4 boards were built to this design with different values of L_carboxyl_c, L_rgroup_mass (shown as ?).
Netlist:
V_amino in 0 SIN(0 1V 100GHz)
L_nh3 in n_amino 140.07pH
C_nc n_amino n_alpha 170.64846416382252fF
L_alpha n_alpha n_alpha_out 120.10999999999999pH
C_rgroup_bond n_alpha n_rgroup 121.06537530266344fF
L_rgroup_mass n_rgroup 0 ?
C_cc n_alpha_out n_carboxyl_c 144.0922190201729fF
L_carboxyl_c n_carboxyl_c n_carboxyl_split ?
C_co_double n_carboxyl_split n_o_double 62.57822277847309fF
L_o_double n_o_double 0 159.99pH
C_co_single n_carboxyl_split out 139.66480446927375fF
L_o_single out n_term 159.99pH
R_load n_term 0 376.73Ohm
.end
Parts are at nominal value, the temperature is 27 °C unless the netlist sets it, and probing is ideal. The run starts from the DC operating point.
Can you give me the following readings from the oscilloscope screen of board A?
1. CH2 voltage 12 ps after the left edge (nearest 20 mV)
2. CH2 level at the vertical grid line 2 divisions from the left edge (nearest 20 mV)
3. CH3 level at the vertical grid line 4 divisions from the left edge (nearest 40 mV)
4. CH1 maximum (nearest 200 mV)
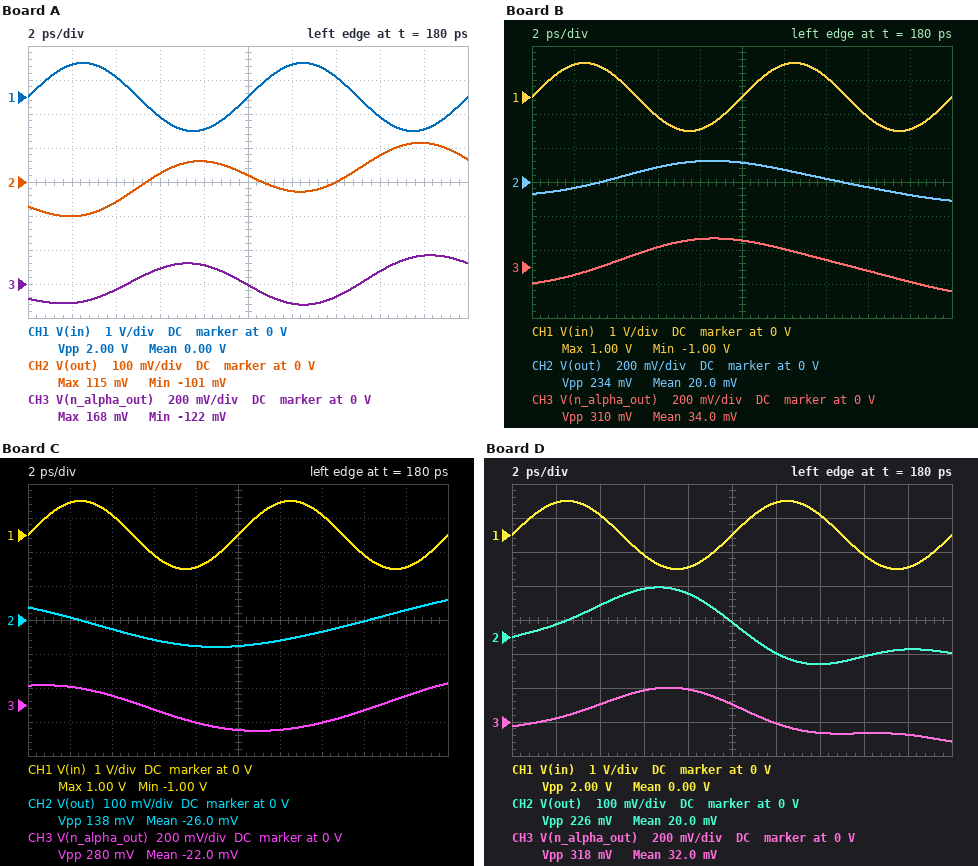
-20 mV
-60 mV
120 mV
1.0 V
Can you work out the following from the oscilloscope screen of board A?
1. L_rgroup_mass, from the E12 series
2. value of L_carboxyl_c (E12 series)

5.6 pH
100 pH
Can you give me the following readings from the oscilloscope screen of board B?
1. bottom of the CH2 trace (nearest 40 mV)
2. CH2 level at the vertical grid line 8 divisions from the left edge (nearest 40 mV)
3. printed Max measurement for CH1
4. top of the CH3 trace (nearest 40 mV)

-120 mV
-40 mV
1.00 V
160 mV
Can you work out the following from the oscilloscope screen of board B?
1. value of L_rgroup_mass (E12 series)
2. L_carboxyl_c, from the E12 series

18 pH
56 pH
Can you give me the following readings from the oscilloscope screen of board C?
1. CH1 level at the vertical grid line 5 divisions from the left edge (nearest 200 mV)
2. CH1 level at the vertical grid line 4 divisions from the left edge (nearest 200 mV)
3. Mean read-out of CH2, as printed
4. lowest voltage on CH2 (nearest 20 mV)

0 V
-1.0 V
-26.0 mV
-80 mV
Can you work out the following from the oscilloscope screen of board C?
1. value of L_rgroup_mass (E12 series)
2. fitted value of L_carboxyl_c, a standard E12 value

22 pH
150 pH
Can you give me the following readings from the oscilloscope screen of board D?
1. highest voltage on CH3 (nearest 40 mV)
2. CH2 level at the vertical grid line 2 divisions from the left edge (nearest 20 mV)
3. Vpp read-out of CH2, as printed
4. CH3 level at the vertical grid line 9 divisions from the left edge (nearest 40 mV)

200 mV
100 mV
226 mV
-80 mV
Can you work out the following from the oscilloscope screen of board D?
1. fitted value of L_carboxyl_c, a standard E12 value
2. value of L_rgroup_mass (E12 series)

47 pH
12 pH
